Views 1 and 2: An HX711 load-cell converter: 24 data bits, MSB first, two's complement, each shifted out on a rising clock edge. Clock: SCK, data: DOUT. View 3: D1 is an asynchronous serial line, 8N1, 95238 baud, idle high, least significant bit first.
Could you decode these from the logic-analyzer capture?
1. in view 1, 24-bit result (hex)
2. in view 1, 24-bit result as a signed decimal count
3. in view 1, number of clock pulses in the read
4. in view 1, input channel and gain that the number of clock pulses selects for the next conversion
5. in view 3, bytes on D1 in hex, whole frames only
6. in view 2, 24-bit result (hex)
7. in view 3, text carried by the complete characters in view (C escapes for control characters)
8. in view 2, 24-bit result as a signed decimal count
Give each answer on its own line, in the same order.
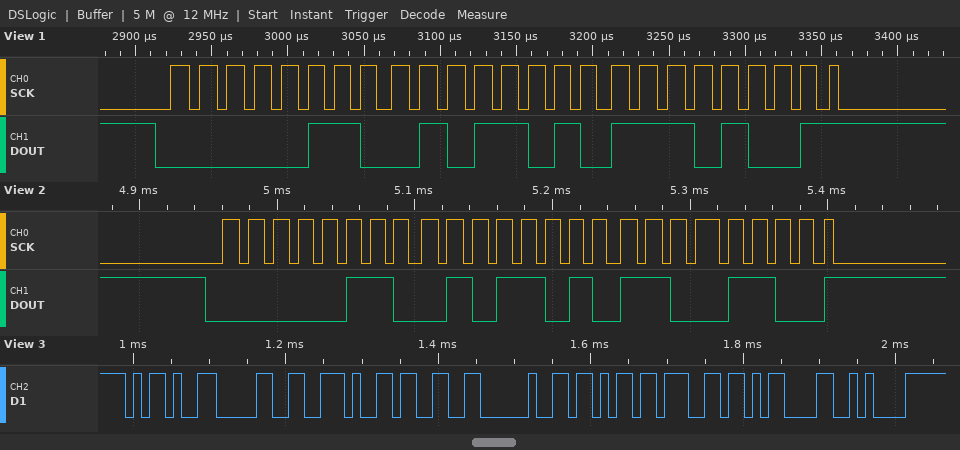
0x065AE9
416489
25
channel A, gain 128
2D 30 2E 33 20 6B 67 0D 0A
0x065ACC
"-0.3 kg\r\n"
416460
